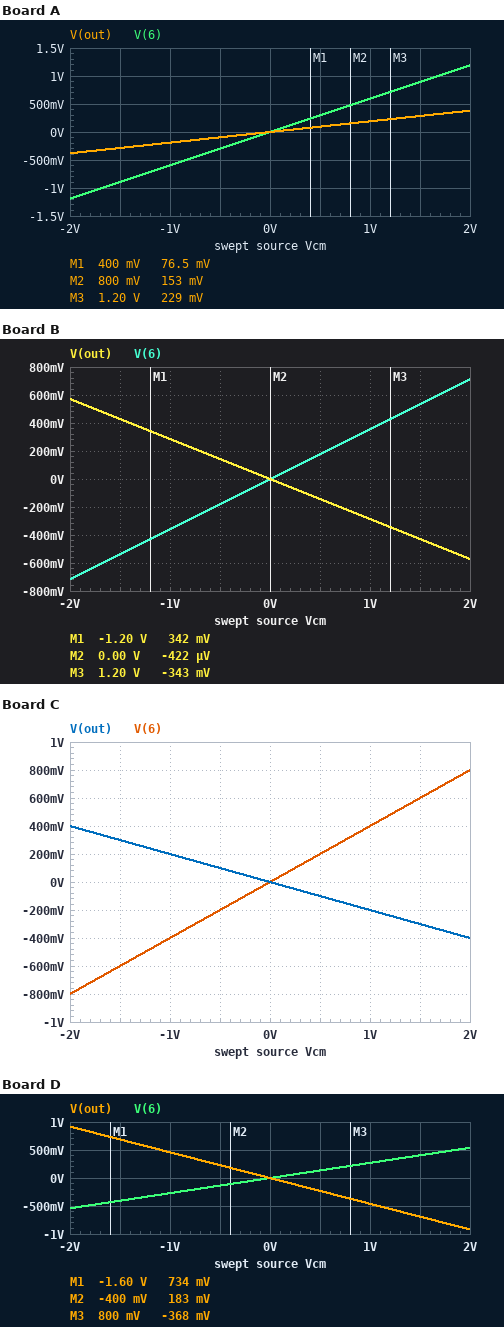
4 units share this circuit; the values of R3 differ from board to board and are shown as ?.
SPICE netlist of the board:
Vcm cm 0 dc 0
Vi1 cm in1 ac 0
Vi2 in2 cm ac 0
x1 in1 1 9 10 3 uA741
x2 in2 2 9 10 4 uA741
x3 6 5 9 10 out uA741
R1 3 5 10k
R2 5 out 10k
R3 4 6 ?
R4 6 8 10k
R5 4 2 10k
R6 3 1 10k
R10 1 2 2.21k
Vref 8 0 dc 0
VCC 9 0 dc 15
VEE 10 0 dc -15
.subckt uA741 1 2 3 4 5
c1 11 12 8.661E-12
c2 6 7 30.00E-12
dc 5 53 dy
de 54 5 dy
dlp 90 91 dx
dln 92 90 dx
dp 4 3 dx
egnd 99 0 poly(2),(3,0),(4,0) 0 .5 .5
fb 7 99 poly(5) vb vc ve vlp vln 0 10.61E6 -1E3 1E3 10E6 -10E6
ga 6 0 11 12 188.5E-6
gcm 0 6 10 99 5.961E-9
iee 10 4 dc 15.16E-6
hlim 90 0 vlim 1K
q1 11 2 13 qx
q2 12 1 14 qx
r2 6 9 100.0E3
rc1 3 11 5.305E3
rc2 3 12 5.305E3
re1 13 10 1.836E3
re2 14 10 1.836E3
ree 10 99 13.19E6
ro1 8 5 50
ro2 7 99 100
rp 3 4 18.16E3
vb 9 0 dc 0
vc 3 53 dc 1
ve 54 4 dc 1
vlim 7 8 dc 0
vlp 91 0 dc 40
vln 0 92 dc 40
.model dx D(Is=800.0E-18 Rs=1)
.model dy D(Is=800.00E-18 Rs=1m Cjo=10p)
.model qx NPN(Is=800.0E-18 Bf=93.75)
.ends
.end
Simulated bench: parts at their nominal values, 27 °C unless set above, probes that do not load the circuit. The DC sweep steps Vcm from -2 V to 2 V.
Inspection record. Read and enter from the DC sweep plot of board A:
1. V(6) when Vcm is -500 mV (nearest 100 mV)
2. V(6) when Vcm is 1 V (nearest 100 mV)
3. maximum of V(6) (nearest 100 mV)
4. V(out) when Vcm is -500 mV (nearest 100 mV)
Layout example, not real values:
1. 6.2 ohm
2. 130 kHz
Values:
1. -300 mV
2. 600 mV
3. 1.2 V
4. -100 mV
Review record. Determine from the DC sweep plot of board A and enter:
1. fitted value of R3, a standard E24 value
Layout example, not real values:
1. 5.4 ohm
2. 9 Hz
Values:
1. 6.8 kΩ
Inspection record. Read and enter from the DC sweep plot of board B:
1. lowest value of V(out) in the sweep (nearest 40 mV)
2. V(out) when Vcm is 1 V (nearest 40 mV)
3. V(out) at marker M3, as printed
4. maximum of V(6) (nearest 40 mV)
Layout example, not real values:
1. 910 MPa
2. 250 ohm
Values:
1. -560 mV
2. -280 mV
3. -343 mV
4. 720 mV
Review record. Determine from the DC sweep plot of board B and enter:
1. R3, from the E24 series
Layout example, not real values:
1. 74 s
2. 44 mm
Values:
1. 18 kΩ
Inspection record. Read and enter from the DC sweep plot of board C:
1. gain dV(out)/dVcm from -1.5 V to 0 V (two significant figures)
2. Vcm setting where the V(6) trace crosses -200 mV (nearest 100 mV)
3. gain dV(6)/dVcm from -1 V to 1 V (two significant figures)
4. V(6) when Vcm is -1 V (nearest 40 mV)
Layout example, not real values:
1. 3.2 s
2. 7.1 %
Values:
1. -0.20 V/V
2. -500 mV
3. 0.40 V/V
4. -400 mV
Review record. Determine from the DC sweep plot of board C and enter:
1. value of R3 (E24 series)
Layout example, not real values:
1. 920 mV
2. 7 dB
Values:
1. 15 kΩ
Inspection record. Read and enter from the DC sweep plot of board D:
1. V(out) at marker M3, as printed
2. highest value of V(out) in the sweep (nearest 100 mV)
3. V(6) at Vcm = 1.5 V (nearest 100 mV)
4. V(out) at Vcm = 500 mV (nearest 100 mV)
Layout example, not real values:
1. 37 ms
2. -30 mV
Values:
1. -368 mV
2. 900 mV
3. 400 mV
4. -200 mV
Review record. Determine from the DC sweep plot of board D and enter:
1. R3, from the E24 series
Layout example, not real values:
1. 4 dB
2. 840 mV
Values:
1. 27 kΩ
